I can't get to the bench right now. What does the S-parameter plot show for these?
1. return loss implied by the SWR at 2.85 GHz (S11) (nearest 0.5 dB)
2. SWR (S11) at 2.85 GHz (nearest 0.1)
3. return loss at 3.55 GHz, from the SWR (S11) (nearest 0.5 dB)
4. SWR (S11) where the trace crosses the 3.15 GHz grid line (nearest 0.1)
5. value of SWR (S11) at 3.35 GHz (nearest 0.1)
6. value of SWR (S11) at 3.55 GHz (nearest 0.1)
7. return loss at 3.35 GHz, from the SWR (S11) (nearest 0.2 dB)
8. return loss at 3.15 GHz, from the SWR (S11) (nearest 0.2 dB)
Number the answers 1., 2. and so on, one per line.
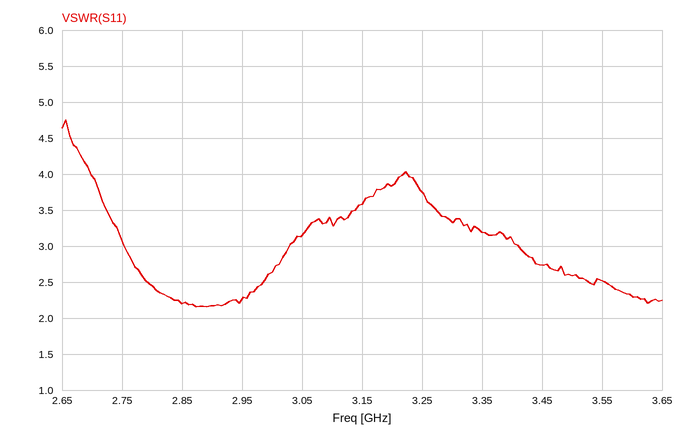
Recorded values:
1. 8.5 dB
2. 2.2
3. 7.5 dB
4. 3.6
5. 3.2
6. 2.5
7. 5.6 dB
8. 5.0 dB
